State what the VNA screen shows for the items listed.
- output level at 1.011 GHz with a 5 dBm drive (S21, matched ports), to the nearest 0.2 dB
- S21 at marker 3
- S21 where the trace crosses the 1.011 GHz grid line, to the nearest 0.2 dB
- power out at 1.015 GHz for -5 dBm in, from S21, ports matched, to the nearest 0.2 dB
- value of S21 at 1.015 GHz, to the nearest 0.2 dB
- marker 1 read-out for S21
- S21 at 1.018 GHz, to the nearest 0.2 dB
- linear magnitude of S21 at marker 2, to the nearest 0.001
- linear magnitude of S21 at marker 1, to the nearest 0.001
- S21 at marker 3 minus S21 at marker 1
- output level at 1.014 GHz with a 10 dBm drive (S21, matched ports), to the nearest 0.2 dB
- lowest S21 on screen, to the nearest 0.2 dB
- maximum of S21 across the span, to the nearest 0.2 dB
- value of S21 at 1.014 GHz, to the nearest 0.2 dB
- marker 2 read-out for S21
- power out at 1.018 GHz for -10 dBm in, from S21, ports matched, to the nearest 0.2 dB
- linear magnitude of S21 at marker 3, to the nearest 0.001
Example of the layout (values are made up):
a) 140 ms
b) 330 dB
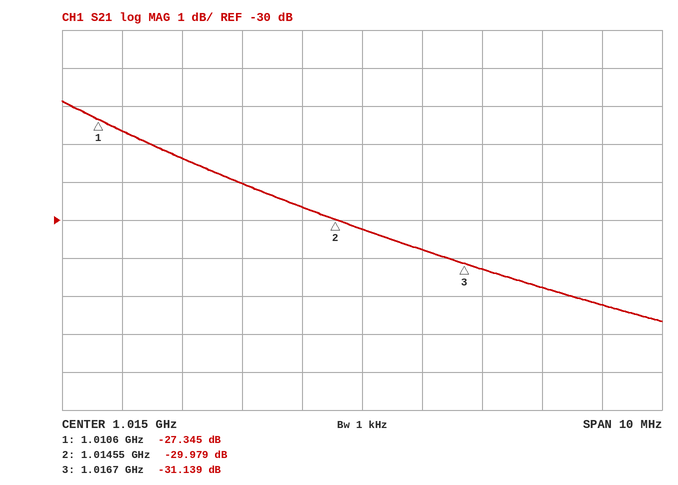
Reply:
a) -22.6 dBm
b) -31.139 dB
c) -27.6 dB
d) -35.2 dBm
e) -30.2 dB
f) -27.345 dB
g) -31.8 dB
h) 0.032
i) 0.043
j) -3.794 dB
k) -19.6 dBm
l) -32.6 dB
m) -26.8 dB
n) -29.6 dB
o) -29.979 dB
p) -41.8 dBm
q) 0.028
